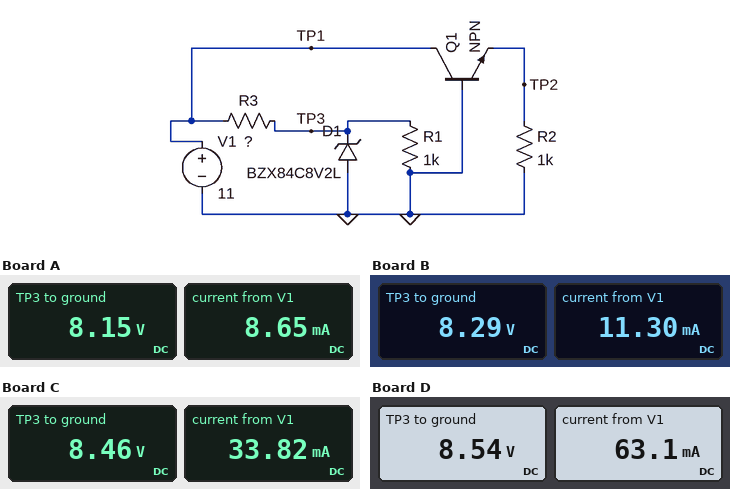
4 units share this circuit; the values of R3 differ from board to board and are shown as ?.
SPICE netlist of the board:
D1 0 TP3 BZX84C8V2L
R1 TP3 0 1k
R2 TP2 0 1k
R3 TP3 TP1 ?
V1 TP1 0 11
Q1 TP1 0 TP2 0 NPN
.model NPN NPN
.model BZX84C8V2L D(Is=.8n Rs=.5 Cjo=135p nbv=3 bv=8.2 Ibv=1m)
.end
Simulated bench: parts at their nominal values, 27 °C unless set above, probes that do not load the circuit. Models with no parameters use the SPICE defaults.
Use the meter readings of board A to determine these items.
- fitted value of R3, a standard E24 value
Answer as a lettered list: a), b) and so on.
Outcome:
a) 330 Ω
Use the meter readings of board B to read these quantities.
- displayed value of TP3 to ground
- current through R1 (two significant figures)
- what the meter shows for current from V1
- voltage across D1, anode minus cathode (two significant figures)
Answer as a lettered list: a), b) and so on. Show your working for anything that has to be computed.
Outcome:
a) 8.29 V
b) (8.29 V) / 1 kΩ = 8.3 mA
c) 11.30 mA
d) 0 V - 8.29 V = -8.3 V
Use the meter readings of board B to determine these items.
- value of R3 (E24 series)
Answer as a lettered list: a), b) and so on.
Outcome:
a) 240 Ω
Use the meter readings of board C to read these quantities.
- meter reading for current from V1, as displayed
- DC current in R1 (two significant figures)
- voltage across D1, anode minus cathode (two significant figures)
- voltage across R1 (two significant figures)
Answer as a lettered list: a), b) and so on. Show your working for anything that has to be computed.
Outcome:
a) 33.82 mA
b) (8.46 V) / 1 kΩ = 8.5 mA
c) 0 V - 8.46 V = -8.5 V
d) 8.46 V = 8.5 V
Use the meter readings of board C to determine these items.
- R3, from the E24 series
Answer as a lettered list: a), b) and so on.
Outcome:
a) 75 Ω
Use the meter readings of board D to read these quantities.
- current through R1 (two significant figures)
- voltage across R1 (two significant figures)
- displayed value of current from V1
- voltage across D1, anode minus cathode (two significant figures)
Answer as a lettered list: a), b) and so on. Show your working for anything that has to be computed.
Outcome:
a) (8.54 V) / 1 kΩ = 8.5 mA
b) 8.54 V = 8.5 V
c) 63.1 mA
d) 0 V - 8.54 V = -8.5 V
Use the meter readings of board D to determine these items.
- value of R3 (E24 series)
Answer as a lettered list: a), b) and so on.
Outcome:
a) 39 Ω
